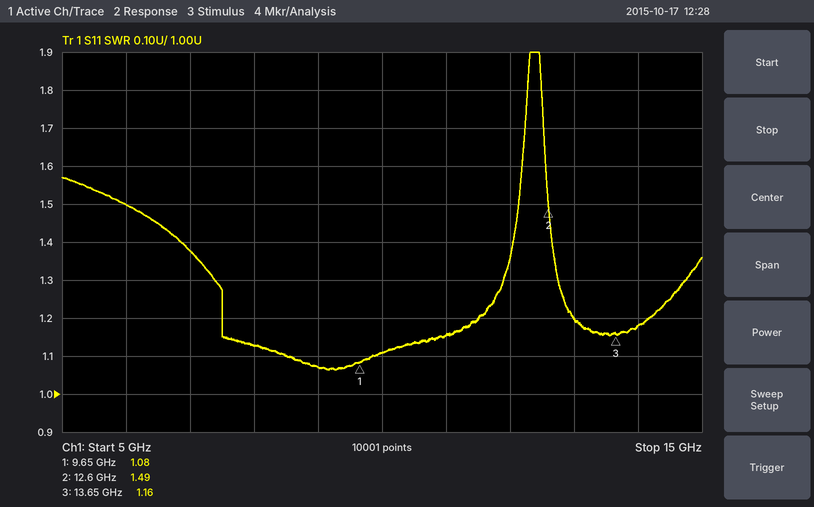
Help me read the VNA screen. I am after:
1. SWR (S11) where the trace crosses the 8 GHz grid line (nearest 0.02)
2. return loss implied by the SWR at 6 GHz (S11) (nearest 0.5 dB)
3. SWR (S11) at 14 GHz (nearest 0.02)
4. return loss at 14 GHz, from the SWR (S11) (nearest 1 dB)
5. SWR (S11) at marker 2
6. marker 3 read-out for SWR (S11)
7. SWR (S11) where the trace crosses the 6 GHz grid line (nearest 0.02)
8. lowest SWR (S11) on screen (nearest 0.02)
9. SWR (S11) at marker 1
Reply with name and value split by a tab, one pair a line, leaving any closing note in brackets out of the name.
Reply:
SWR (S11) where the trace crosses the 8 GHz grid line	1.12
return loss implied by the SWR at 6 GHz (S11)	14.0 dB
SWR (S11) at 14 GHz	1.18
return loss at 14 GHz, from the SWR (S11)	22 dB
SWR (S11) at marker 2	1.49
marker 3 read-out for SWR	1.16
SWR (S11) where the trace crosses the 6 GHz grid line	1.50
lowest SWR (S11) on screen	1.06
SWR (S11) at marker 1	1.08
